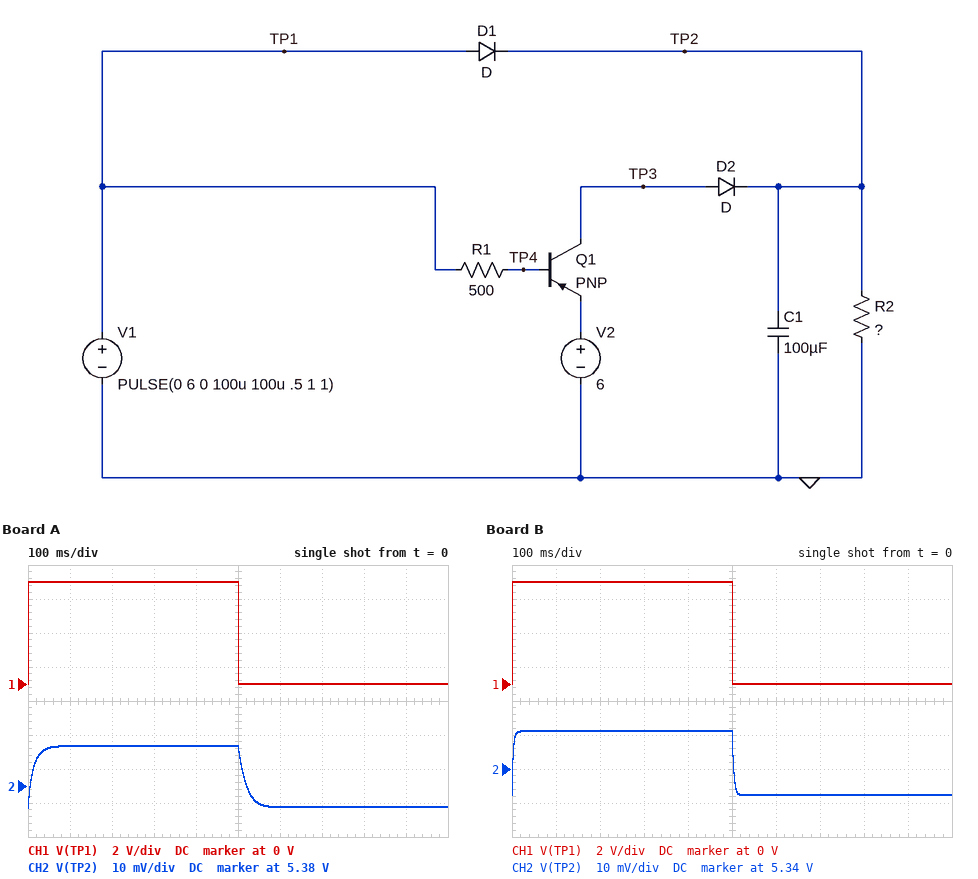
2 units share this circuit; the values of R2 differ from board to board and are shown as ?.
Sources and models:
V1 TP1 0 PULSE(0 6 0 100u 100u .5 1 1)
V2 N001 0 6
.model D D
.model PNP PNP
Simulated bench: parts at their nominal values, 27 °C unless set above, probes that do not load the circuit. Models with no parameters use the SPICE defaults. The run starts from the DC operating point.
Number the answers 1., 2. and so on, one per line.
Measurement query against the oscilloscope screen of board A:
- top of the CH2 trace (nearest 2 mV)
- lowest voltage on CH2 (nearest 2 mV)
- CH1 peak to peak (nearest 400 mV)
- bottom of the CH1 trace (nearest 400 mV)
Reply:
1. 5.392 V
2. 5.374 V
3. 6.0 V
4. 0 V
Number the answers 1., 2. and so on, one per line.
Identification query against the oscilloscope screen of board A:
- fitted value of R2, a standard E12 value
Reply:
1. 33 kΩ
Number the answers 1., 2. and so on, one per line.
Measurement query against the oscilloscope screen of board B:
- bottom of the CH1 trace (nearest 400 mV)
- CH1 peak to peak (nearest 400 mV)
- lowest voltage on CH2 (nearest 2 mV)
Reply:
1. 0 V
2. 6.0 V
3. 5.332 V
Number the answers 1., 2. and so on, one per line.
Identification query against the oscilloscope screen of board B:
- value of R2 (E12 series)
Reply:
1. 6.8 kΩ
